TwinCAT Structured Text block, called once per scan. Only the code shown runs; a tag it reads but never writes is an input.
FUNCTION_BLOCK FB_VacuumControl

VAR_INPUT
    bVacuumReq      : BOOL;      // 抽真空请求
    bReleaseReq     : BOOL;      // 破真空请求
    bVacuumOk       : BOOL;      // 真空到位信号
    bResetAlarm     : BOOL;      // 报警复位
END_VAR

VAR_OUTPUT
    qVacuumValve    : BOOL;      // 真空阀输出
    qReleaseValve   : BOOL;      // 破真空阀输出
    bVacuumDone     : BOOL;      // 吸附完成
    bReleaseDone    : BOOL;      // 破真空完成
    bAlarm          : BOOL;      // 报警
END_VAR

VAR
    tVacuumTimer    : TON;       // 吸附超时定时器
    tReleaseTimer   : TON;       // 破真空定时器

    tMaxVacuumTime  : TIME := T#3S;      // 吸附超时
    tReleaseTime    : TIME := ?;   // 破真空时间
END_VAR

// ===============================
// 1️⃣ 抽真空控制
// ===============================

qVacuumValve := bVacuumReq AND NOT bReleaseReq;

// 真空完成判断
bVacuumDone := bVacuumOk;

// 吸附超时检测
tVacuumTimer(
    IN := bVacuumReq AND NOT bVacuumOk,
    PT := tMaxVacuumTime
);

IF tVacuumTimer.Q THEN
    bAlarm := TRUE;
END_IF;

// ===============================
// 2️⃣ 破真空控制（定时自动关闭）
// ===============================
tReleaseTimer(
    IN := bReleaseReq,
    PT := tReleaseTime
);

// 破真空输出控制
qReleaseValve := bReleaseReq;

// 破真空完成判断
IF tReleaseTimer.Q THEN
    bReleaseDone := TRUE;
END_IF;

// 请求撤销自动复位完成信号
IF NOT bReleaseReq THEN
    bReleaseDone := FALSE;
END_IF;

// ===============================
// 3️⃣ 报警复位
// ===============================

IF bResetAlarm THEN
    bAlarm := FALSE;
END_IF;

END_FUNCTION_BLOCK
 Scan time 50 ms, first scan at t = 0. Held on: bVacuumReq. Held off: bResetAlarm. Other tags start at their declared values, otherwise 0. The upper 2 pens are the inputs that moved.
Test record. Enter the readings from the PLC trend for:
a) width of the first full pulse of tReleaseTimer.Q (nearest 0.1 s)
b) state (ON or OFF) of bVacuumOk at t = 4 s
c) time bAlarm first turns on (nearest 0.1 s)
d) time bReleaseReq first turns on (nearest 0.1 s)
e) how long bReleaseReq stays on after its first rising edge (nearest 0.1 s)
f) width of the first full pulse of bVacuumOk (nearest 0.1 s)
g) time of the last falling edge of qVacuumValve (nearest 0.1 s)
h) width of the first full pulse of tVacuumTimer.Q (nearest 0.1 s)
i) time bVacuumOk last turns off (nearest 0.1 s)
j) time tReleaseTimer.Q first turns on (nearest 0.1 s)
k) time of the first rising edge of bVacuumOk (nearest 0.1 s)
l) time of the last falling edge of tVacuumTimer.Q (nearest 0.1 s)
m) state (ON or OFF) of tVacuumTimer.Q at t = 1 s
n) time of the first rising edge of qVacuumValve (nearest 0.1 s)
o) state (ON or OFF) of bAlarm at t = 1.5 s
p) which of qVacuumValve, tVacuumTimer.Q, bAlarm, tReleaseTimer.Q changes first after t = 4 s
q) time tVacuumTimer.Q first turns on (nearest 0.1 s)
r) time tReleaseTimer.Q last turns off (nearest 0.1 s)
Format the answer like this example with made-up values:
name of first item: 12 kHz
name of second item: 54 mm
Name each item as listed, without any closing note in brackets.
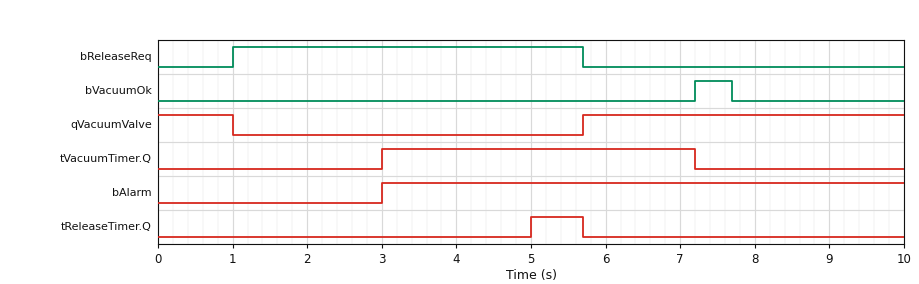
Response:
width of the first full pulse of tReleaseTimer.Q: 0.7 s
state (ON or OFF) of bVacuumOk at t = 4 s: OFF
time bAlarm first turns on: 3.0 s
time bReleaseReq first turns on: 1.0 s
how long bReleaseReq stays on after its first rising edge: 4.7 s
width of the first full pulse of bVacuumOk: 0.5 s
time of the last falling edge of qVacuumValve: 1.0 s
width of the first full pulse of tVacuumTimer.Q: 4.2 s
time bVacuumOk last turns off: 7.7 s
time tReleaseTimer.Q first turns on: 5.0 s
time of the first rising edge of bVacuumOk: 7.2 s
time of the last falling edge of tVacuumTimer.Q: 7.2 s
state (ON or OFF) of tVacuumTimer.Q at t = 1 s: OFF
time of the first rising edge of qVacuumValve: 5.7 s
state (ON or OFF) of bAlarm at t = 1.5 s: OFF
which of qVacuumValve, tVacuumTimer.Q, bAlarm, tReleaseTimer.Q changes first after t = 4 s: tReleaseTimer.Q
time tVacuumTimer.Q first turns on: 3.0 s
time tReleaseTimer.Q last turns off: 5.7 s
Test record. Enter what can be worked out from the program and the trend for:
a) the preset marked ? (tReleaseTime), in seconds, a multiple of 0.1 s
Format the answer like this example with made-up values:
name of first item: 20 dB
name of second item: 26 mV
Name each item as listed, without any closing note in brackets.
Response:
the preset marked ? (tReleaseTime), in seconds, a multiple of 0.1 s: 4.0 s
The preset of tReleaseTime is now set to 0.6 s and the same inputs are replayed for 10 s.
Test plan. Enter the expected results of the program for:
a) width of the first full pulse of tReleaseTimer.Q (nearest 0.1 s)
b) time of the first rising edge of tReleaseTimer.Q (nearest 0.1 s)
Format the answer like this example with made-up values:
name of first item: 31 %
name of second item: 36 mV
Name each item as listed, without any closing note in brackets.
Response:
width of the first full pulse of tReleaseTimer.Q: 4.1 s
time of the first rising edge of tReleaseTimer.Q: 1.6 s
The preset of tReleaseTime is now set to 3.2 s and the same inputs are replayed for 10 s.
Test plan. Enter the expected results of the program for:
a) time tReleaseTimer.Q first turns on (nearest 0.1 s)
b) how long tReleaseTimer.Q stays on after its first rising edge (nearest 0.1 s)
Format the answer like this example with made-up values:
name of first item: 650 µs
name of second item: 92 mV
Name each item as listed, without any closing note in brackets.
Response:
time tReleaseTimer.Q first turns on: 4.2 s
how long tReleaseTimer.Q stays on after its first rising edge: 1.5 s
